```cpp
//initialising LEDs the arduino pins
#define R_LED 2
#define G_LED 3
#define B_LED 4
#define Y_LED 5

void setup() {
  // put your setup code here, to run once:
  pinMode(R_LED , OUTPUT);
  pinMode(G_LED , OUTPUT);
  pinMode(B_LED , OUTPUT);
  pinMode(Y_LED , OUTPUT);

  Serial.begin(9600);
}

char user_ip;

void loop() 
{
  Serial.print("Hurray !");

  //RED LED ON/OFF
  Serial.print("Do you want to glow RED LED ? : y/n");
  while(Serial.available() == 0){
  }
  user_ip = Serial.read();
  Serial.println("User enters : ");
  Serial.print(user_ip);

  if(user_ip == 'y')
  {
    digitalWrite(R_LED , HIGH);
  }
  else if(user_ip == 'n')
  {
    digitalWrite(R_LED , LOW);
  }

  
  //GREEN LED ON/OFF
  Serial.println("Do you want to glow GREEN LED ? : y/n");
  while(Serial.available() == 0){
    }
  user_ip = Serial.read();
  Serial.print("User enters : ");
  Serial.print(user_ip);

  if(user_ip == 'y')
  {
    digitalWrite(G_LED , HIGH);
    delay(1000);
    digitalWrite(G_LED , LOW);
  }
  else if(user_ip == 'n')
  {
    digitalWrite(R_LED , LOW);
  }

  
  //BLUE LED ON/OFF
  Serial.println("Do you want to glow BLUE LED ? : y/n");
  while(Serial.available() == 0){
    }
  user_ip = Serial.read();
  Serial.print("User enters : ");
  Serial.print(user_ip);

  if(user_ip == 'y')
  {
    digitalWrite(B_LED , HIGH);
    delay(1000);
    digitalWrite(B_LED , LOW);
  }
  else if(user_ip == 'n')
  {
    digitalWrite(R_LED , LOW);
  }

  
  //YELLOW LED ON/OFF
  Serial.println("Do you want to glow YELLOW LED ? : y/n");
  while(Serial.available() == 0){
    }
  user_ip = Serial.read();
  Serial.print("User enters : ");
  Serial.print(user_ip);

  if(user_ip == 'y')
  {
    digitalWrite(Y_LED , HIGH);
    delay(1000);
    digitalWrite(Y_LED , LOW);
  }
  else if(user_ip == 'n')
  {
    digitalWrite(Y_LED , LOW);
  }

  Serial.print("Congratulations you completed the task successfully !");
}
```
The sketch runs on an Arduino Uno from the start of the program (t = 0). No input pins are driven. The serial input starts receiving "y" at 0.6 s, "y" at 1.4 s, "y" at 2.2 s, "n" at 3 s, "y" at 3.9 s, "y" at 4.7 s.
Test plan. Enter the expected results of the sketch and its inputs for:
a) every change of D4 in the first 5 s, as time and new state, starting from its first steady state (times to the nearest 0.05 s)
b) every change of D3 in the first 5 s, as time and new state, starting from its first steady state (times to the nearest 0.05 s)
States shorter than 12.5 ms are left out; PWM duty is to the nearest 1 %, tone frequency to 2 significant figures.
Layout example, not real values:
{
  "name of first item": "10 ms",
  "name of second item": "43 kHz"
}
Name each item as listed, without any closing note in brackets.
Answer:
{
  "every change of D4 in the first 5 s, as time and new state, starting from its first steady state": "0 s low; 2.4 s high; 3.4 s low",
  "every change of D3 in the first 5 s, as time and new state, starting from its first steady state": "0 s low; 1.4 s high; 2.4 s low; 4.7 s high"
}
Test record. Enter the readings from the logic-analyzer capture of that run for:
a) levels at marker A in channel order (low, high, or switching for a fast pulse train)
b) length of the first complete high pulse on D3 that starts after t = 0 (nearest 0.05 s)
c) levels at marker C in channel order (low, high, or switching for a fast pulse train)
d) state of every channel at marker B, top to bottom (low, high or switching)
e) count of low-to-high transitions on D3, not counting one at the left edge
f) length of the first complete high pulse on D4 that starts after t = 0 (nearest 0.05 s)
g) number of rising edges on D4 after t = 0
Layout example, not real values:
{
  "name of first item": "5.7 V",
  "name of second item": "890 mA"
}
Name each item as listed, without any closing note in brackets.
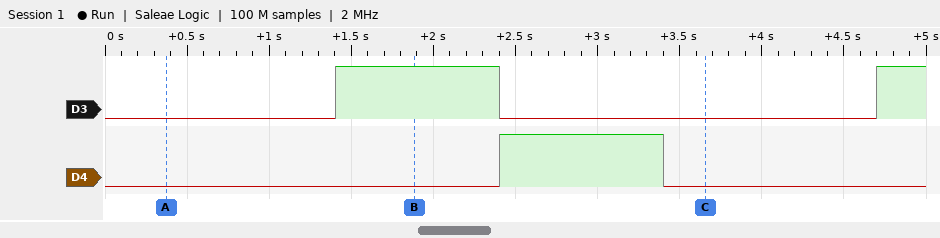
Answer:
{
  "levels at marker A in channel order": "D3 low, D4 low",
  "length of the first complete high pulse on D3 that starts after t = 0": "1.00 s",
  "levels at marker C in channel order": "D3 low, D4 low",
  "state of every channel at marker B, top to bottom": "D3 high, D4 low",
  "count of low-to-high transitions on D3, not counting one at the left edge": "2",
  "length of the first complete high pulse on D4 that starts after t = 0": "1.00 s",
  "number of rising edges on D4 after t = 0": "1"
}
